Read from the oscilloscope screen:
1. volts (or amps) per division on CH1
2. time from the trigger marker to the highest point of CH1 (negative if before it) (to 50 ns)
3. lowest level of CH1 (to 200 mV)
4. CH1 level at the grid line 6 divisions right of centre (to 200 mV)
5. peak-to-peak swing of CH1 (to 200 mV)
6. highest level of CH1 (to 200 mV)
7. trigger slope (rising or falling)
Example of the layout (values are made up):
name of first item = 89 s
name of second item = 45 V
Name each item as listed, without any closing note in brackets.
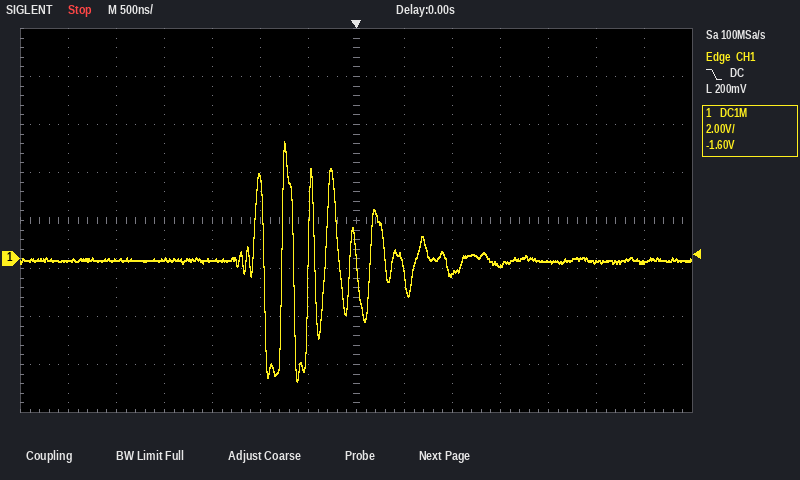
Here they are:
volts (or amps) per division on CH1 = 2 V
time from the trigger marker to the highest point of CH1 (negative if before it) = -750 ns
lowest level of CH1 = -5.2 V
CH1 level at the grid line 6 divisions right of centre = -200 mV
peak-to-peak swing of CH1 = 10.0 V
highest level of CH1 = 4.8 V
trigger slope = falling
